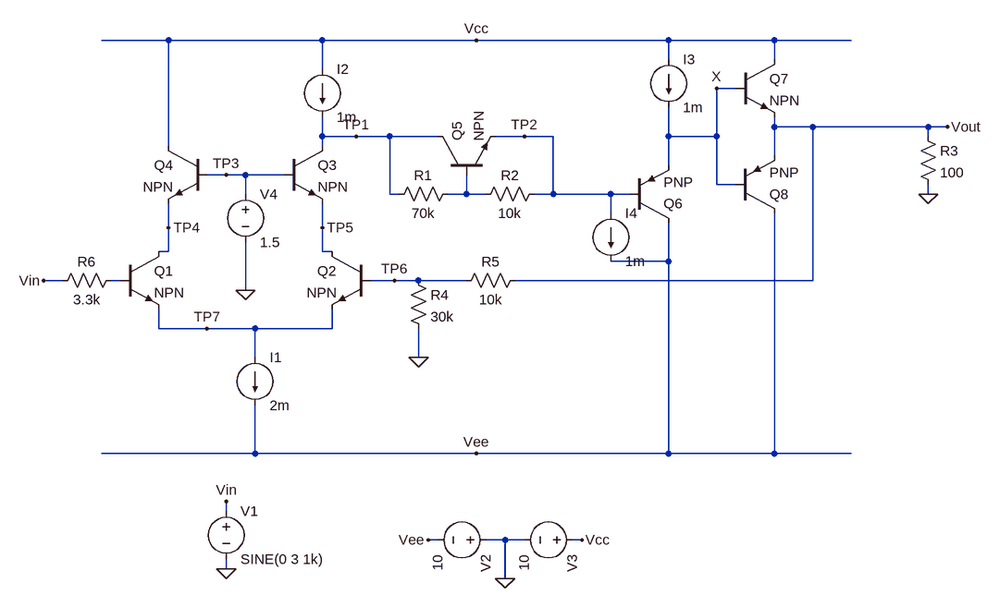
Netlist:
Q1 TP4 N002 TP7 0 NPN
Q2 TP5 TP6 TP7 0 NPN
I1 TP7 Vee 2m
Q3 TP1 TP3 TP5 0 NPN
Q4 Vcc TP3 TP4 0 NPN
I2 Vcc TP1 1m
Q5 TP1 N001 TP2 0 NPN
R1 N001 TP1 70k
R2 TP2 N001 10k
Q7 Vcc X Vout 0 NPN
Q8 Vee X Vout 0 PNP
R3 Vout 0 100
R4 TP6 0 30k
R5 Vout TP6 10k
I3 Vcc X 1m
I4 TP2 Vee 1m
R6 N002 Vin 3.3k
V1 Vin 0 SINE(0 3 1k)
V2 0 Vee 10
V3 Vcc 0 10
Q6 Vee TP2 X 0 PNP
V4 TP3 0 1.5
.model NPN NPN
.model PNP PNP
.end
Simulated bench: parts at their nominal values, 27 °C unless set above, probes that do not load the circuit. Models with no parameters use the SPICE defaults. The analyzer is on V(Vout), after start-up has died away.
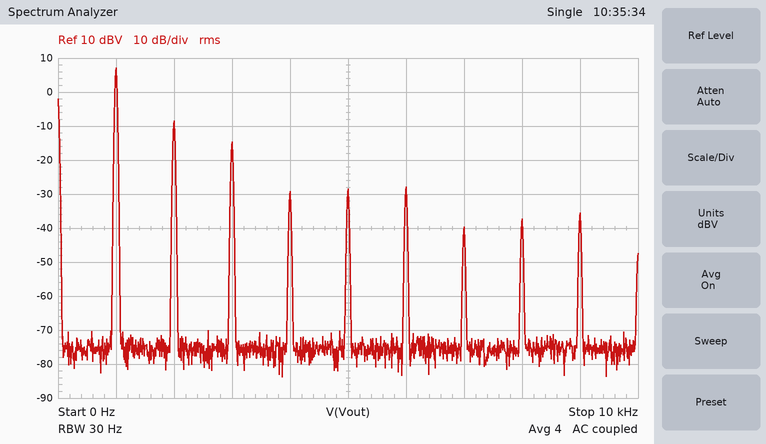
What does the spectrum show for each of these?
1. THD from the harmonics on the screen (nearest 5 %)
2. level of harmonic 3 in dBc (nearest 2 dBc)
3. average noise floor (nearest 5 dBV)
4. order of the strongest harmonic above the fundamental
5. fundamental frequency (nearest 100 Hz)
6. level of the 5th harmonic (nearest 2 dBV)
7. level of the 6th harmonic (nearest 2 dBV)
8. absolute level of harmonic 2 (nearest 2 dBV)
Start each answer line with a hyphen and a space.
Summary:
- 20 %
- -22 dBc
- -75 dBV
- 2
- 1.0 kHz
- -28 dBV
- -28 dBV
- -8 dBV
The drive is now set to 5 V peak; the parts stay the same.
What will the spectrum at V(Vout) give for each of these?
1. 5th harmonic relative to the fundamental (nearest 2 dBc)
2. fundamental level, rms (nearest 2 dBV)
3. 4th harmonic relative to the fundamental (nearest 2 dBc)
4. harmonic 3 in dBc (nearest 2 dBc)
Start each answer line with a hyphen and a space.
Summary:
- -28 dBc
- 8 dBV
- -22 dBc
- -14 dBc
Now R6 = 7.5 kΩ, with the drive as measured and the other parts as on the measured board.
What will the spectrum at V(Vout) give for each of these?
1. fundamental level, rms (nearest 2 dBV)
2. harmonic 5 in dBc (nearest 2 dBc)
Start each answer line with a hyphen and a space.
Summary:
- 8 dBV
- -38 dBc
